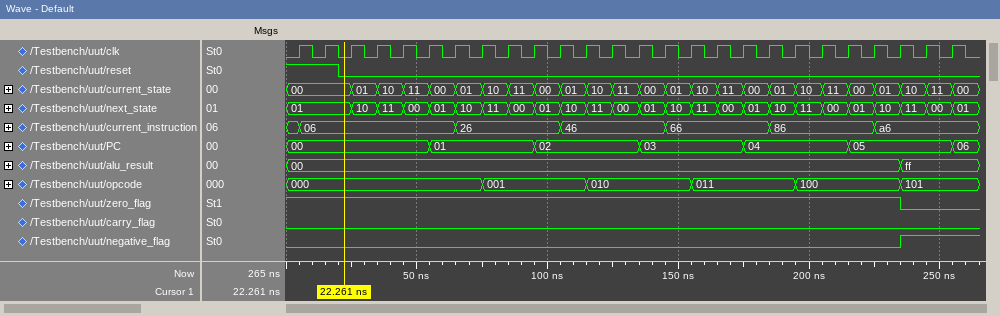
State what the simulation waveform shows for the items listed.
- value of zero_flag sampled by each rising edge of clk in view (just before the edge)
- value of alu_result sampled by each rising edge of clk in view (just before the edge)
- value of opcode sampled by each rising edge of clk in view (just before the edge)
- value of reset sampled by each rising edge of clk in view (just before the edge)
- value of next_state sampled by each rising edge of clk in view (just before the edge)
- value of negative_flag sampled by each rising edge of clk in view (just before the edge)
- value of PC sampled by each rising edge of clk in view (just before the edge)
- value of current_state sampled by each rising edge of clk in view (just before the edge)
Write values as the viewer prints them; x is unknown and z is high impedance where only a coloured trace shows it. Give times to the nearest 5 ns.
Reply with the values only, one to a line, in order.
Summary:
1 1 1 1 1 1 1 1 1 1 1 1 1 1 1 1 1 1 1 1 1 1 1 1 0 0
00, 00, 00, 00, 00, 00, 00, 00, 00, 00, 00, 00, 00, 00, 00, 00, 00, 00, 00, 00, 00, 00, 00, 00, ff, ff
000, 000, 000, 000, 000, 000, 000, 000, 001, 001, 001, 001, 010, 010, 010, 010, 011, 011, 011, 011, 100, 100, 100, 100, 101, 101
1 1 0 0 0 0 0 0 0 0 0 0 0 0 0 0 0 0 0 0 0 0 0 0 0 0
01, 01, 01, 10, 11, 00, 01, 10, 11, 00, 01, 10, 11, 00, 01, 10, 11, 00, 01, 10, 11, 00, 01, 10, 11, 00
0 0 0 0 0 0 0 0 0 0 0 0 0 0 0 0 0 0 0 0 0 0 0 0 1 1
00, 00, 00, 00, 00, 00, 01, 01, 01, 01, 02, 02, 02, 02, 03, 03, 03, 03, 04, 04, 04, 04, 05, 05, 05, 05
00, 00, 00, 01, 10, 11, 00, 01, 10, 11, 00, 01, 10, 11, 00, 01, 10, 11, 00, 01, 10, 11, 00, 01, 10, 11
